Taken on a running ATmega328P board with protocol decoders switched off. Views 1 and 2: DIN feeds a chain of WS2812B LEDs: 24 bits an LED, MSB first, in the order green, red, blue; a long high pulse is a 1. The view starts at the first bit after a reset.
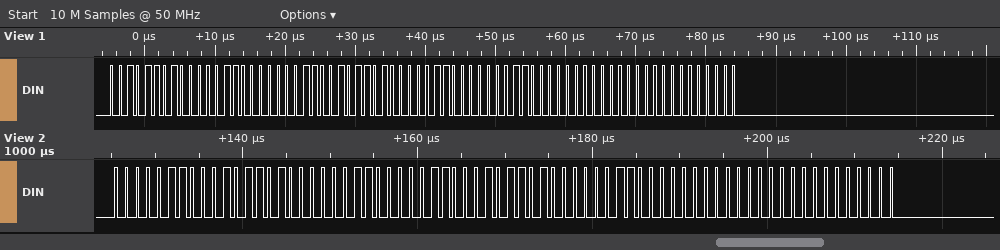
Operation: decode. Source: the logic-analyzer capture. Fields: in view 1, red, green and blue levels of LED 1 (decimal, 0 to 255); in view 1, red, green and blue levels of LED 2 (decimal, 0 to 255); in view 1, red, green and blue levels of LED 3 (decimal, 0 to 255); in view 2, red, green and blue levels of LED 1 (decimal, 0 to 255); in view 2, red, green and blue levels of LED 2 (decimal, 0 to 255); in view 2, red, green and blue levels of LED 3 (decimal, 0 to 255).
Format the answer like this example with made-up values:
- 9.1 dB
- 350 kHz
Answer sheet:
- 6, 45, 3
- 6, 45, 3
- 0, 0, 0
- 45, 6, 3
- 45, 6, 3
- 0, 0, 0
